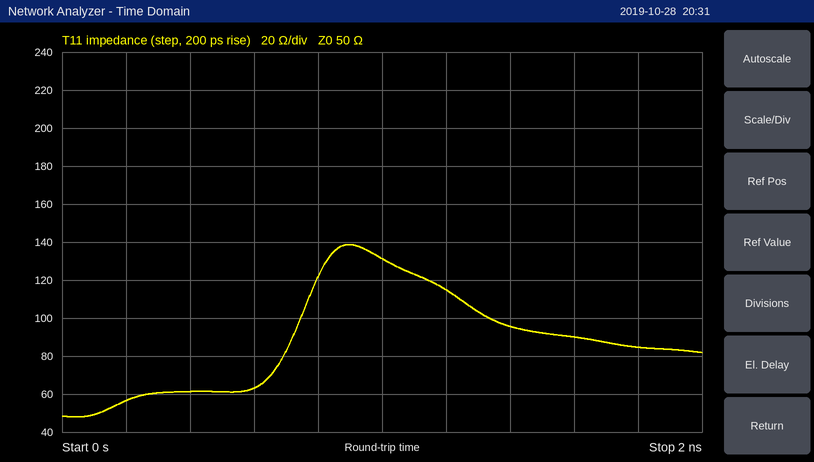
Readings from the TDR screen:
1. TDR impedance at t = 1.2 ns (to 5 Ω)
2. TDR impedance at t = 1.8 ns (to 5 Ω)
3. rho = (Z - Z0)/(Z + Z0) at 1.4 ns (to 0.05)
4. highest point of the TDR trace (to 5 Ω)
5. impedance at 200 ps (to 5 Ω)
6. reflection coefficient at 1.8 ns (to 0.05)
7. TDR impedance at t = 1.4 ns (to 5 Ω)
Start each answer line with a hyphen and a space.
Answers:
- 115 Ω
- 85 Ω
- +0.30
- 140 Ω
- 55 Ω
- +0.25
- 95 Ω
